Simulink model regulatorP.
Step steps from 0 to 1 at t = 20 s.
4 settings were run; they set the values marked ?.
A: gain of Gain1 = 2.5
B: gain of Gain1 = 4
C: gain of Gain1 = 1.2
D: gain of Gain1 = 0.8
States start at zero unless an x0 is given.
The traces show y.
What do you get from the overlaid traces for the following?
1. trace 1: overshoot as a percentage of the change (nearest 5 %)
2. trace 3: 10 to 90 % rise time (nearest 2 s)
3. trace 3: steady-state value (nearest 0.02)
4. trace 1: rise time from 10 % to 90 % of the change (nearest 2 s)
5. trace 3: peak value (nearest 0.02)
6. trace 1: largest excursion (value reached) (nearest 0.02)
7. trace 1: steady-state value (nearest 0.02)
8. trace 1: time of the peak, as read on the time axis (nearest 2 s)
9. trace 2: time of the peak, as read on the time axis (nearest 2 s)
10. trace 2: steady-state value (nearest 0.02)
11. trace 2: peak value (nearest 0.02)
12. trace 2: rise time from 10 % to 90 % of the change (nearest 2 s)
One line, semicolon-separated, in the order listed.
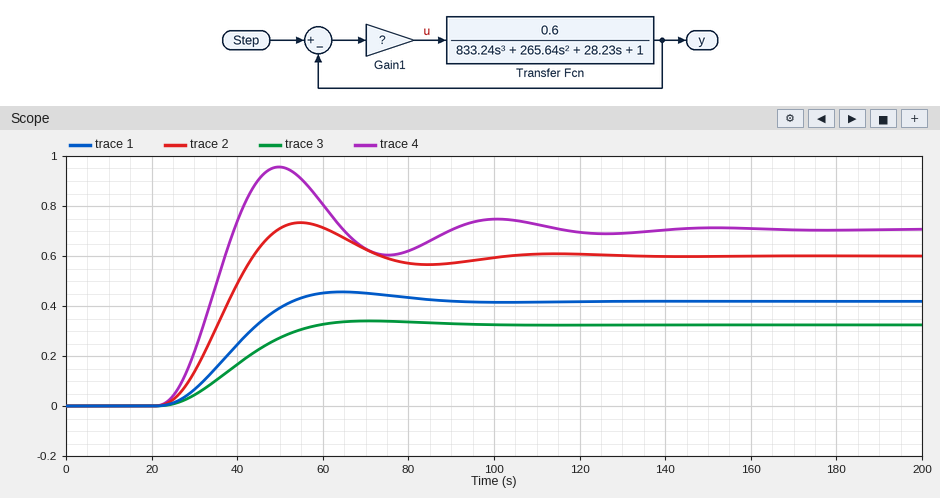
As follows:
10 %; 24 s; 0.32; 20 s; 0.34; 0.46; 0.42; 64 s; 54 s; 0.60; 0.74; 14 s
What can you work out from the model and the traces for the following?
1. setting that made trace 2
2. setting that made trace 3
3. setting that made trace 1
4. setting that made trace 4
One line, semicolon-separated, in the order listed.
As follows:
A; D; C; B
